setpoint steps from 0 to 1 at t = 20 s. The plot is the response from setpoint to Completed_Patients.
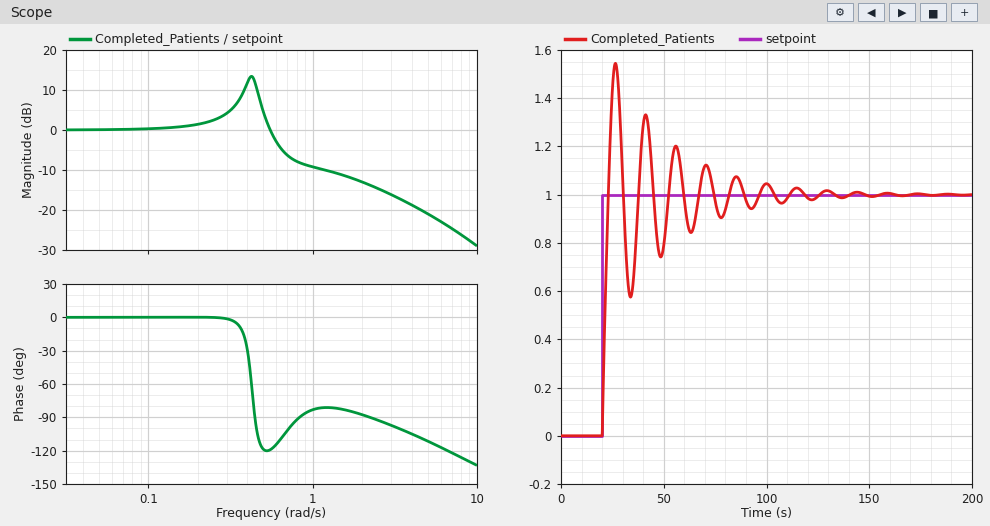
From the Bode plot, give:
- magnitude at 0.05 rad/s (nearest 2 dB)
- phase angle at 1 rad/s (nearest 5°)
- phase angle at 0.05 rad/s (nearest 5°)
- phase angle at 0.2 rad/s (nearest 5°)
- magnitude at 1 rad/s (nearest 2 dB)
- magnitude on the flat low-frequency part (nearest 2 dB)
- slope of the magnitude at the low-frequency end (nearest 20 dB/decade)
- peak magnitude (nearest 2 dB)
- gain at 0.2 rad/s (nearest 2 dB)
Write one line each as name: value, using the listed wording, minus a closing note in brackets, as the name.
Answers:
magnitude at 0.05 rad/s: 0 dB
phase angle at 1 rad/s: -85°
phase angle at 0.05 rad/s: 0°
phase angle at 0.2 rad/s: 0°
magnitude at 1 rad/s: -10 dB
magnitude on the flat low-frequency part: 0 dB
slope of the magnitude at the low-frequency end: 0 dB/decade
peak magnitude: 14 dB
gain at 0.2 rad/s: 2 dB
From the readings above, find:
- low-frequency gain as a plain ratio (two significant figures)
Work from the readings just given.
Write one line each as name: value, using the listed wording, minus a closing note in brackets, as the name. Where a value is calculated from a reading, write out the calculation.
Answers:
low-frequency gain as a plain ratio: 10^(0 / 20) = 1.0
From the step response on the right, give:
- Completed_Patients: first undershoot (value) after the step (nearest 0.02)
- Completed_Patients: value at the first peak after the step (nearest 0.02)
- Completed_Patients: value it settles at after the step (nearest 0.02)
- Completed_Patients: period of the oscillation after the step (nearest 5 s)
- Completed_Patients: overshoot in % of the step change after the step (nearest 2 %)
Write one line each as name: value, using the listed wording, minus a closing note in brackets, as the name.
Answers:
Completed_Patients: first undershoot (value) after the step: 0.58
Completed_Patients: value at the first peak after the step: 1.54
Completed_Patients: value it settles at after the step: 1.00
Completed_Patients: period of the oscillation after the step: 15 s
Completed_Patients: overshoot in % of the step change after the step: 54 %
